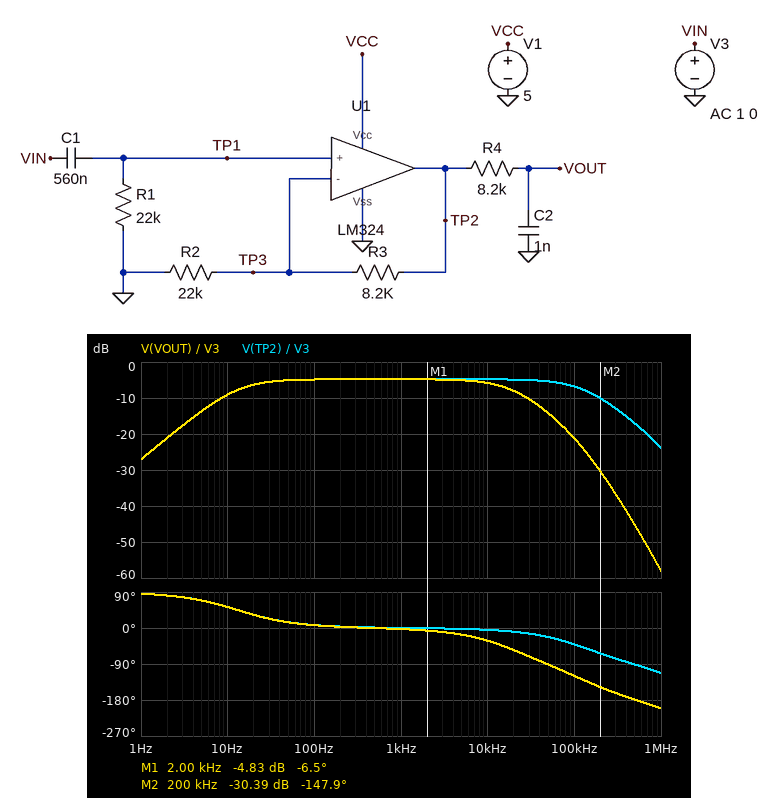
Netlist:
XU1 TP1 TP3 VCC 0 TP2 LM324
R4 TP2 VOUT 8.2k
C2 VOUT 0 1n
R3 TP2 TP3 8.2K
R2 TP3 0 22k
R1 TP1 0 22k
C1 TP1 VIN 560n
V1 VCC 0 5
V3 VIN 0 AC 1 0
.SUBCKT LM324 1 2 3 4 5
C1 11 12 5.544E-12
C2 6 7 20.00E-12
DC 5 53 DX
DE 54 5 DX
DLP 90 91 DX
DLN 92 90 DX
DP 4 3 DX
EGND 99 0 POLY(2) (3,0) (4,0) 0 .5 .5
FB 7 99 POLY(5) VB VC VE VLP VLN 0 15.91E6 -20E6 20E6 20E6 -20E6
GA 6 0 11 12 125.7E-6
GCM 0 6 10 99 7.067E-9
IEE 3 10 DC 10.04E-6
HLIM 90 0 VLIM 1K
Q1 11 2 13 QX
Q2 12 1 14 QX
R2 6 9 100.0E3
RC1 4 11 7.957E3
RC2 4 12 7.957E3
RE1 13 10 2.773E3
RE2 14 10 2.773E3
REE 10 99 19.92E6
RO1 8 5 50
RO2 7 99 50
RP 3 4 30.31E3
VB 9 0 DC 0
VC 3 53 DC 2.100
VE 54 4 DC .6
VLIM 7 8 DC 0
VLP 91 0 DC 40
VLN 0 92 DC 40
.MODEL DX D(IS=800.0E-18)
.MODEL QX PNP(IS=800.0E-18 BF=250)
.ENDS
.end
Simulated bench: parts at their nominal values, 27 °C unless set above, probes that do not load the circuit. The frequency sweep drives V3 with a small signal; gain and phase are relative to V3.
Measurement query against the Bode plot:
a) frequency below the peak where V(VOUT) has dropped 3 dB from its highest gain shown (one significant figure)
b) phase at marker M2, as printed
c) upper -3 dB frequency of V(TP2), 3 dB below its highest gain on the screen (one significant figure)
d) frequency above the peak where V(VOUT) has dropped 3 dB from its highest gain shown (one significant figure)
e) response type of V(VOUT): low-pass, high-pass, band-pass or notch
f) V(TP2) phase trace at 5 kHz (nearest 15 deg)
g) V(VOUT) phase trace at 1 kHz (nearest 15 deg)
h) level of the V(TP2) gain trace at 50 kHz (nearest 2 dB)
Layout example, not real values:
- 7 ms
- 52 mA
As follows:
- 10 Hz
- -147.9 deg
- 100 kHz
- 20 kHz
- band-pass
- 0 deg
- 0 deg
- -6 dB
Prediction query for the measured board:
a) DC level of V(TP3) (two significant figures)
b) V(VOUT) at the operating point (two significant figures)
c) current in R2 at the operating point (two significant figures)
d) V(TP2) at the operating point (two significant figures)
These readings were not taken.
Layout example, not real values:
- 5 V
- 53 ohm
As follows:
- 26 mV
- 35 mV
- 1.2 µA
- 35 mV
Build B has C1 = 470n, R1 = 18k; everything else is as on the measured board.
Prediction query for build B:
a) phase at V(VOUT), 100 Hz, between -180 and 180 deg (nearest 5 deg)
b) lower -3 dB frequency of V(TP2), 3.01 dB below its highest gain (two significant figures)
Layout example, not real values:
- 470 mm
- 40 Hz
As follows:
- 10 deg
- 19 Hz
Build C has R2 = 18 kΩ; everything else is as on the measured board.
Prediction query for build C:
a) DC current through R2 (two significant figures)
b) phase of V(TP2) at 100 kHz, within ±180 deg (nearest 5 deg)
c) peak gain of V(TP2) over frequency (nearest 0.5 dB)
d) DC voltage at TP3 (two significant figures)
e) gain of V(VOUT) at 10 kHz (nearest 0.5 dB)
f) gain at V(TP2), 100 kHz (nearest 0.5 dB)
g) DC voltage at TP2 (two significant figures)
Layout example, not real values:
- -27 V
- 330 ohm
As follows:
- 1.4 µA
- -40 deg
- -4.5 dB
- 25 mV
- -5.5 dB
- -6.5 dB
- 36 mV
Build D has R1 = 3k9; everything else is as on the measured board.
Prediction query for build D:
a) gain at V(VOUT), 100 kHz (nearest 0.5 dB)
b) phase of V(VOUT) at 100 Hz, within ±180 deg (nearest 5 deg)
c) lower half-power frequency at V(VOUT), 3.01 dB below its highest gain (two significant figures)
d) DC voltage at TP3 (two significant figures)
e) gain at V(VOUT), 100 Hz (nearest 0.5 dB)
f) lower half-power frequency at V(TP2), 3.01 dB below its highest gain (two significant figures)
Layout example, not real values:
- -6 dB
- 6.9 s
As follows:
- -21.5 dB
- 35 deg
- 72 Hz
- 25 mV
- -6.5 dB
- 73 Hz
